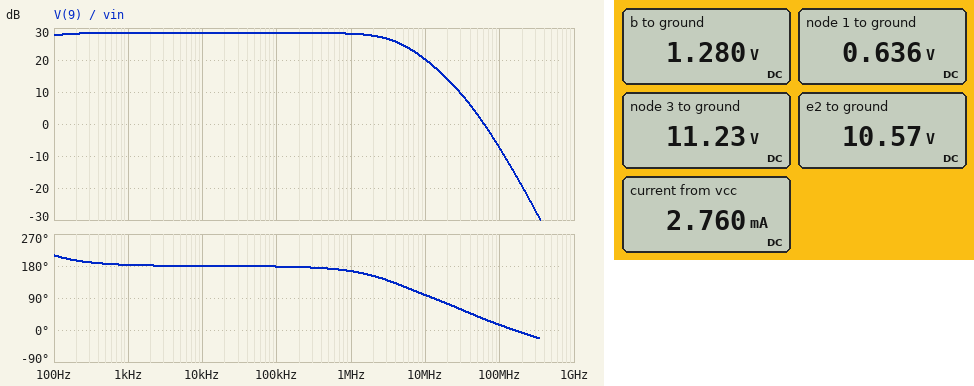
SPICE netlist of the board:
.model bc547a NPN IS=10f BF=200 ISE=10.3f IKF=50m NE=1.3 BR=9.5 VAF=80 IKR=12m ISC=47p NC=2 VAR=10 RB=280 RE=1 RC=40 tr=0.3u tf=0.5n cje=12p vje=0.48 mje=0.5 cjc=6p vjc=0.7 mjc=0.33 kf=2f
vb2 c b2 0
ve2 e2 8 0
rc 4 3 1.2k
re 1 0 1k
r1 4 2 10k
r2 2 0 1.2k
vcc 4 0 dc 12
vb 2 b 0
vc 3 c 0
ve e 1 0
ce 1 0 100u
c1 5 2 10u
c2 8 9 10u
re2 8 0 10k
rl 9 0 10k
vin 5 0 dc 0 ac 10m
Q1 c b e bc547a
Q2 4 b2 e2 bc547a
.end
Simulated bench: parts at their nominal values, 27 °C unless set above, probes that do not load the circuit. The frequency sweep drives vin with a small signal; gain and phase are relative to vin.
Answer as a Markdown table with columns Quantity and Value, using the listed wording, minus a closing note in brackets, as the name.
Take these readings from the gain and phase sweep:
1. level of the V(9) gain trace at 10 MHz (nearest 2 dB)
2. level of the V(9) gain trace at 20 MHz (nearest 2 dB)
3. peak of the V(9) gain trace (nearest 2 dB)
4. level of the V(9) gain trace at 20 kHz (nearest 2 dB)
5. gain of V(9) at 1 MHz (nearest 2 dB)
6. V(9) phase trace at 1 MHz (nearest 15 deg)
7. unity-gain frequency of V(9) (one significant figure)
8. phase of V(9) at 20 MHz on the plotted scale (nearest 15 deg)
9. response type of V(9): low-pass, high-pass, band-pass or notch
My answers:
| Quantity | Value |
|---|---|
| level of the V(9) gain trace at 10 MHz | 20 dB |
| level of the V(9) gain trace at 20 MHz | 14 dB |
| peak of the V(9) gain trace | 28 dB |
| level of the V(9) gain trace at 20 kHz | 28 dB |
| gain of V(9) at 1 MHz | 28 dB |
| V(9) phase trace at 1 MHz | 165 deg |
| unity-gain frequency of V(9) | 60 MHz |
| phase of V(9) at 20 MHz on the plotted scale | 75 deg |
| response type of V(9): low-pass, high-pass, band-pass or notch | low-pass |
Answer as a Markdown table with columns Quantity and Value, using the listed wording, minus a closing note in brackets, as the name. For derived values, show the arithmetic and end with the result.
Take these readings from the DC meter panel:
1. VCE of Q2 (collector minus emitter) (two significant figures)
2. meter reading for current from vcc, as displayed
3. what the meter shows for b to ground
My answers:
| Quantity | Value |
|---|---|
| VCE of Q2 (collector minus emitter) | 12 V - 10.57 V = 1.4 V |
| meter reading for current from vcc, as displayed | 2.760 mA |
| what the meter shows for b to ground | 1.280 V |
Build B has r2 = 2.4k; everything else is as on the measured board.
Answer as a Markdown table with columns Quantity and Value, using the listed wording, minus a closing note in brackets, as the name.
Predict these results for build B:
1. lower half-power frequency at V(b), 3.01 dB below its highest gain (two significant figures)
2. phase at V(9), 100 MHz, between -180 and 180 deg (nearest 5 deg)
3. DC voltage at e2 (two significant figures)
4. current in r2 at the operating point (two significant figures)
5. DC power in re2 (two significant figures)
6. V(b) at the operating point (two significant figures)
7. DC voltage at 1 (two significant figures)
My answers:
| Quantity | Value |
|---|---|
| lower half-power frequency at V(b), 3.01 dB below its highest gain | 9.1 Hz |
| phase at V(9), 100 MHz, between -180 and 180 deg | 25 deg |
| DC voltage at e2 | 9.4 V |
| current in r2 at the operating point | 960 µA |
| DC power in re2 | 8.8 mW |
| V(b) at the operating point | 2.3 V |
| DC voltage at 1 | 1.6 V |
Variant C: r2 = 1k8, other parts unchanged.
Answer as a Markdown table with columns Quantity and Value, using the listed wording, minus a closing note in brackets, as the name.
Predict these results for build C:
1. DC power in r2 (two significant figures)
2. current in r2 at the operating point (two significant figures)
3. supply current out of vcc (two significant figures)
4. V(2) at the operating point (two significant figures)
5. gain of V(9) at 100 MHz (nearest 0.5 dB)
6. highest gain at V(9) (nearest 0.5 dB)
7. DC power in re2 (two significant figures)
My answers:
| Quantity | Value |
|---|---|
| DC power in r2 | 1.8 mW |
| current in r2 at the operating point | 1.0 mA |
| supply current out of vcc | 3.2 mA |
| V(2) at the operating point | 1.8 V |
| gain of V(9) at 100 MHz | -4.5 dB |
| highest gain at V(9) | 33.0 dB |
| DC power in re2 | 9.9 mW |
